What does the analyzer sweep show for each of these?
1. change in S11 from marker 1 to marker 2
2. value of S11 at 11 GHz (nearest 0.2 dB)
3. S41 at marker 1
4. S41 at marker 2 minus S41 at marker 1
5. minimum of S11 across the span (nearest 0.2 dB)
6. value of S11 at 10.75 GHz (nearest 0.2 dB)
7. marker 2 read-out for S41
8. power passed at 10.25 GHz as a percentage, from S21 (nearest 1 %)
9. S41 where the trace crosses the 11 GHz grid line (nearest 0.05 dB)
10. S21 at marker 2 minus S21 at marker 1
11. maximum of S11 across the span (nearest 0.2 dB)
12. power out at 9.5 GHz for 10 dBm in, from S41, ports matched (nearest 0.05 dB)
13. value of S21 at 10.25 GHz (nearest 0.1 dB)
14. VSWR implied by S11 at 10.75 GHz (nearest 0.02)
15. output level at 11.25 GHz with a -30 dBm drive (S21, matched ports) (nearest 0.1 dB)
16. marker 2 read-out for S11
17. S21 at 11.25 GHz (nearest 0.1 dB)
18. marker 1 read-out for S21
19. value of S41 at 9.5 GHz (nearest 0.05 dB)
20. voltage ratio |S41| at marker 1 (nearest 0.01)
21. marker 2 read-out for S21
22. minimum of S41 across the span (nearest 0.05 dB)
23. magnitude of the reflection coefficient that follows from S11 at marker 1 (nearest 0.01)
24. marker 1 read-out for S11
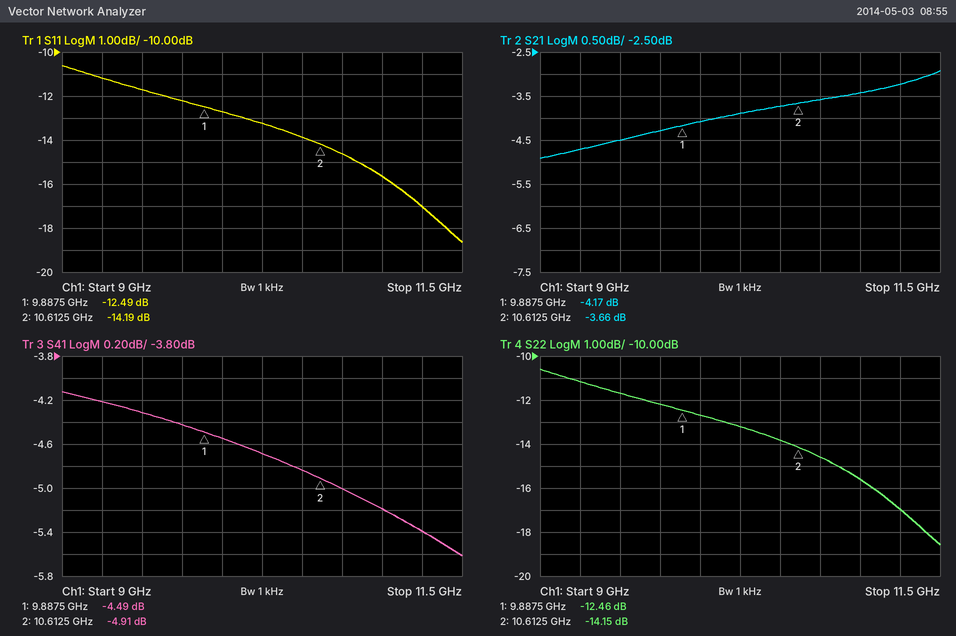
-1.70 dB
-15.6 dB
-4.49 dB
-0.42 dB
-18.6 dB
-14.6 dB
-4.91 dB
41 %
-5.20 dB
0.51 dB
-10.6 dB
5.70 dBm
-3.9 dB
1.46
-33.2 dBm
-14.19 dB
-3.2 dB
-4.17 dB
-4.30 dB
0.60
-3.66 dB
-5.60 dB
0.24
-12.49 dB
